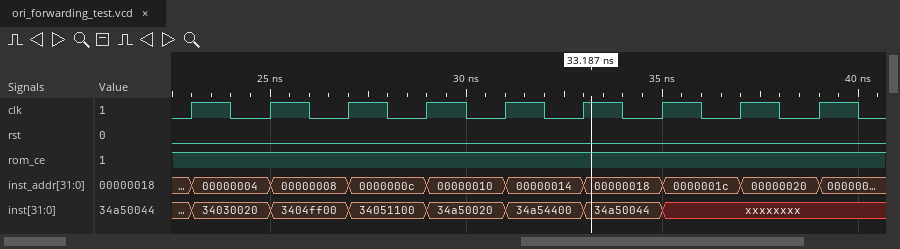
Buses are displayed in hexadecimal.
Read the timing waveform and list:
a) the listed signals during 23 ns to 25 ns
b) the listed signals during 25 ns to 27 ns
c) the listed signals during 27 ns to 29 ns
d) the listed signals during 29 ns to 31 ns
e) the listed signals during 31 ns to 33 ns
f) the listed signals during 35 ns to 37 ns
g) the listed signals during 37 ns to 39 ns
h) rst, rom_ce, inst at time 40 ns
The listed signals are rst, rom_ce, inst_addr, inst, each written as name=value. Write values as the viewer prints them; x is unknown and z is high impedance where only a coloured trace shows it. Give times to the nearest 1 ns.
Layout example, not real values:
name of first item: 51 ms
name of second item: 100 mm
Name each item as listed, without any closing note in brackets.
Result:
the listed signals during 23 ns to 25 ns: rst=0, rom_ce=1, inst_addr=00000004, inst=34030020
the listed signals during 25 ns to 27 ns: rst=0, rom_ce=1, inst_addr=00000008, inst=3404ff00
the listed signals during 27 ns to 29 ns: rst=0, rom_ce=1, inst_addr=0000000c, inst=34051100
the listed signals during 29 ns to 31 ns: rst=0, rom_ce=1, inst_addr=00000010, inst=34a50020
the listed signals during 31 ns to 33 ns: rst=0, rom_ce=1, inst_addr=00000014, inst=34a54400
the listed signals during 35 ns to 37 ns: rst=0, rom_ce=1, inst_addr=0000001c, inst=xxxxxxxx
the listed signals during 37 ns to 39 ns: rst=0, rom_ce=1, inst_addr=00000020, inst=xxxxxxxx
rst, rom_ce, inst at time 40 ns: rst=0, rom_ce=1, inst=xxxxxxxx
